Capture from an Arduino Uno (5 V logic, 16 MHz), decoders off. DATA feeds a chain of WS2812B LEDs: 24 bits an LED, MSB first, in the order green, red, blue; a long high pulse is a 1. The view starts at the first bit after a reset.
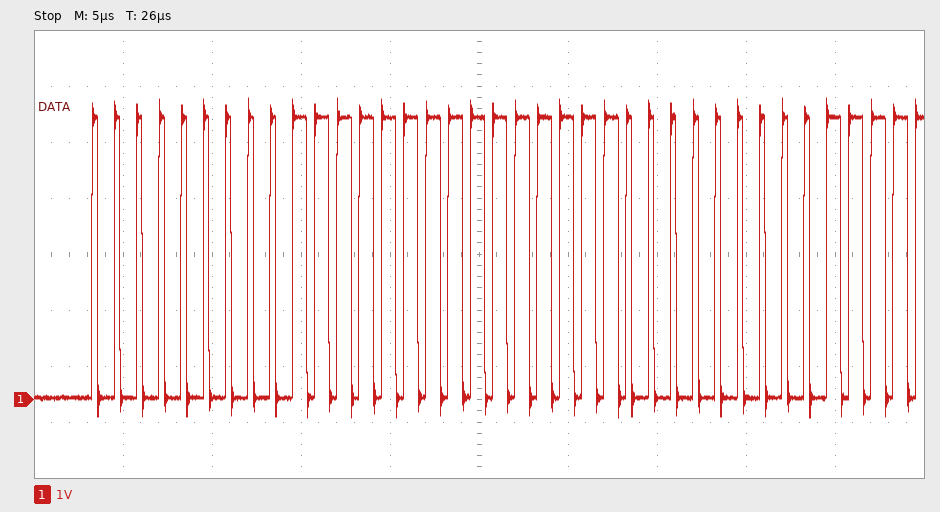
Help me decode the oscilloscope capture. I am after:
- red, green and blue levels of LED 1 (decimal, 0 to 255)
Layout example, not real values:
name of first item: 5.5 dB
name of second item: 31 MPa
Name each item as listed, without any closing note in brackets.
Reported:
red, green and blue levels of LED 1: 127, 0, 255
